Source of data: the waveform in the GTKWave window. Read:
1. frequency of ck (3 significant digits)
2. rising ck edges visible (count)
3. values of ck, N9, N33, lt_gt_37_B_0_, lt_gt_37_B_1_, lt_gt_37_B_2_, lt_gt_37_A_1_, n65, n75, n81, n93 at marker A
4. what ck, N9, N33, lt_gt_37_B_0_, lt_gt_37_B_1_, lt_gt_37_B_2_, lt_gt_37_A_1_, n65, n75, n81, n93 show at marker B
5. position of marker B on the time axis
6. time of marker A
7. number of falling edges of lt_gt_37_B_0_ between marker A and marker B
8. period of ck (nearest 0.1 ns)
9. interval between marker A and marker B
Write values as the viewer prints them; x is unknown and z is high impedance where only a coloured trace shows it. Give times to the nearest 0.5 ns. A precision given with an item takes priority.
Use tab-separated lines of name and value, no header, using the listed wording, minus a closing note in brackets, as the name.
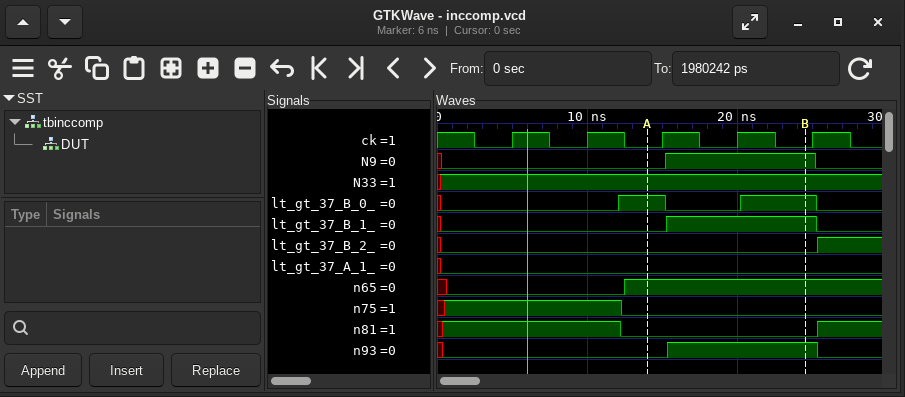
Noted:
frequency of ck	200 MHz
rising ck edges visible	5
values of ck, N9, N33, lt_gt_37_B_0_, lt_gt_37_B_1_, lt_gt_37_B_2_, lt_gt_37_A_1_, n65, n75, n81, n93 at marker A	ck=0, N9=0, N33=1, lt_gt_37_B_0_=1, lt_gt_37_B_1_=0, lt_gt_37_B_2_=0, lt_gt_37_A_1_=0, n65=1, n75=0, n81=0, n93=0
what ck, N9, N33, lt_gt_37_B_0_, lt_gt_37_B_1_, lt_gt_37_B_2_, lt_gt_37_A_1_, n65, n75, n81, n93 show at marker B	ck=0, N9=1, N33=1, lt_gt_37_B_0_=1, lt_gt_37_B_1_=1, lt_gt_37_B_2_=0, lt_gt_37_A_1_=0, n65=1, n75=0, n81=0, n93=1
position of marker B on the time axis	24.5 ns
time of marker A	14 ns
number of falling edges of lt_gt_37_B_0_ between marker A and marker B	1
period of ck	5 ns
interval between marker A and marker B	10.5 ns
